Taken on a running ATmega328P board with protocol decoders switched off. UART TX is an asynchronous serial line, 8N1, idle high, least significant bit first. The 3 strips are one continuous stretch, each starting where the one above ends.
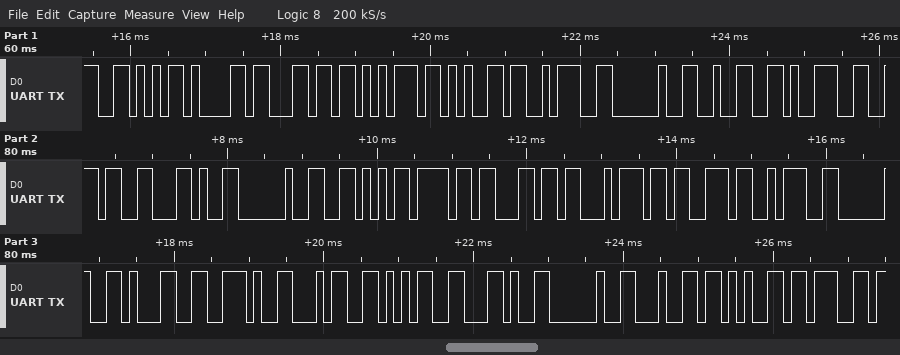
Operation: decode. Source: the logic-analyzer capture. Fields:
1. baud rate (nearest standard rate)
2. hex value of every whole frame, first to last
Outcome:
9600 baud
0x56 0x61 0x6C 0x75 0x65 0x3A 0x20 0x32 0x39 0x36 0x2C 0x20 0x56 0x6F 0x6C 0x74 0x73 0x3A 0x20 0x31 0x2E 0x34 0x35 0x2C 0x20 0x64 0x65 0x67
